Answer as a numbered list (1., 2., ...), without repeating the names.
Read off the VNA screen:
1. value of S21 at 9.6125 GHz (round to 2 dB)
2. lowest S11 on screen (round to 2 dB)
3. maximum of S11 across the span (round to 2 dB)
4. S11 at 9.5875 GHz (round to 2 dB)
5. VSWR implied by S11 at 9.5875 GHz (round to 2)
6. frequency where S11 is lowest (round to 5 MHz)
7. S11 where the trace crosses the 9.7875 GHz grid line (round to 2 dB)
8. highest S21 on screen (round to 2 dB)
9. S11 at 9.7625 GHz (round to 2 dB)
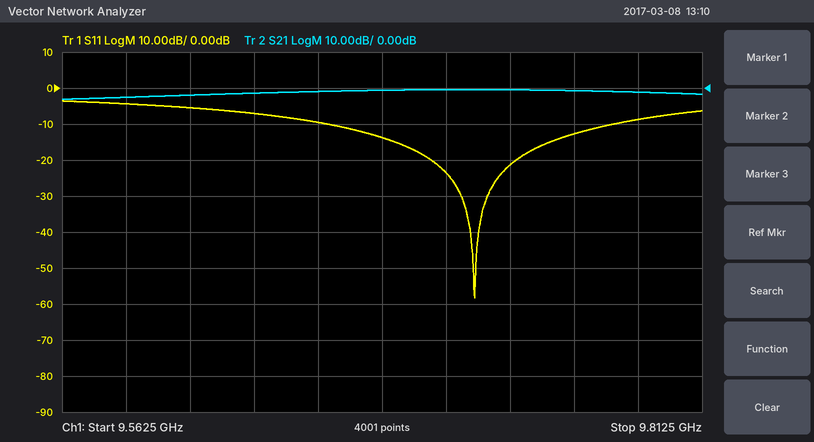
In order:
1. -2 dB
2. -58 dB
3. -4 dB
4. -4 dB
5. 4
6. 9.725 GHz
7. -8 dB
8. 0 dB
9. -12 dB
